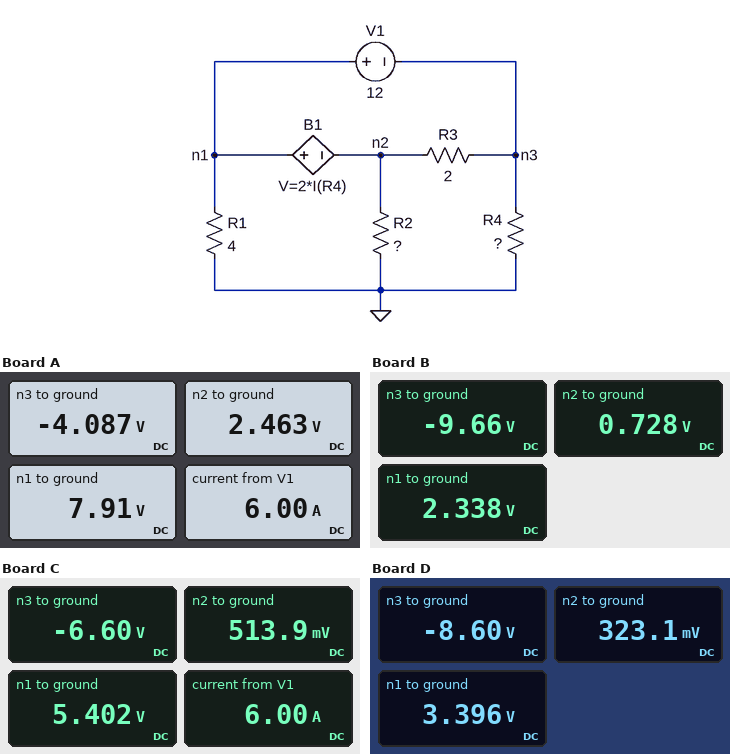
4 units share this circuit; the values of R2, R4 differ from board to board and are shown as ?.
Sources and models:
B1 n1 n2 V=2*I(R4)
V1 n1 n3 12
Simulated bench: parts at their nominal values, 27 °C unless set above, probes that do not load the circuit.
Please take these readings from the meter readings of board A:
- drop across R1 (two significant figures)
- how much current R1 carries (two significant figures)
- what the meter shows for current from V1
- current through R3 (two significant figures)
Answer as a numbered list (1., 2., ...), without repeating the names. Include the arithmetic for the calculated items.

1. 7.91 V = 7.9 V
2. (7.91 V) / 4 Ω = 2.0 A
3. 6.00 A
4. (2.463 V - (-4.087 V)) / 2 Ω = 3.3 A
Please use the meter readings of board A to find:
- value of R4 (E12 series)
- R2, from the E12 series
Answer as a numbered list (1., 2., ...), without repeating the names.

1. 1.5 Ω
2. 3.3 Ω
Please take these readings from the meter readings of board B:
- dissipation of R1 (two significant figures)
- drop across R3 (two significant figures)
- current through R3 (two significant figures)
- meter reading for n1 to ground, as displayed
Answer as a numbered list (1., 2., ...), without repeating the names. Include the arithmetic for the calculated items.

1. (2.338 V)^2 / 4 Ω = 1.4 W
2. 728 mV - (-9.66 V) = 10 V
3. (728 mV - (-9.66 V)) / 2 Ω = 5.2 A
4. 2.338 V
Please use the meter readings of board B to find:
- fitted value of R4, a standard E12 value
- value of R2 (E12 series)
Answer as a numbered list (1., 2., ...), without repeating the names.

1. 12 Ω
2. 3.3 Ω
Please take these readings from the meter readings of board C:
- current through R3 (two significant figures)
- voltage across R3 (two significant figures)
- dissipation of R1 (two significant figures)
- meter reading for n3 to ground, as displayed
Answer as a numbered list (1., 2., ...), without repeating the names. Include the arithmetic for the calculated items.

1. (513.9 mV - (-6.6 V)) / 2 Ω = 3.6 A
2. 513.9 mV - (-6.6 V) = 7.1 V
3. (5.402 V)^2 / 4 Ω = 7.3 W
4. -6.60 V
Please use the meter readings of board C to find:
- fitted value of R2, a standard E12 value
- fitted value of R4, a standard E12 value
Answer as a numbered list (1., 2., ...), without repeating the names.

1. 0.47 Ω
2. 2.7 Ω
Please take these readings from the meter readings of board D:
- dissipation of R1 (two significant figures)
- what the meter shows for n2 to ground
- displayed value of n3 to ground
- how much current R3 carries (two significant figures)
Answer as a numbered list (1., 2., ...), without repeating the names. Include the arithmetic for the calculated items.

1. (3.396 V)^2 / 4 Ω = 2.9 W
2. 323.1 mV
3. -8.60 V
4. (323.1 mV - (-8.6 V)) / 2 Ω = 4.5 A
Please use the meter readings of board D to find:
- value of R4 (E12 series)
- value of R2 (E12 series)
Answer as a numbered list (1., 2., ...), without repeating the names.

1. 5.6 Ω
2. 0.47 Ω
